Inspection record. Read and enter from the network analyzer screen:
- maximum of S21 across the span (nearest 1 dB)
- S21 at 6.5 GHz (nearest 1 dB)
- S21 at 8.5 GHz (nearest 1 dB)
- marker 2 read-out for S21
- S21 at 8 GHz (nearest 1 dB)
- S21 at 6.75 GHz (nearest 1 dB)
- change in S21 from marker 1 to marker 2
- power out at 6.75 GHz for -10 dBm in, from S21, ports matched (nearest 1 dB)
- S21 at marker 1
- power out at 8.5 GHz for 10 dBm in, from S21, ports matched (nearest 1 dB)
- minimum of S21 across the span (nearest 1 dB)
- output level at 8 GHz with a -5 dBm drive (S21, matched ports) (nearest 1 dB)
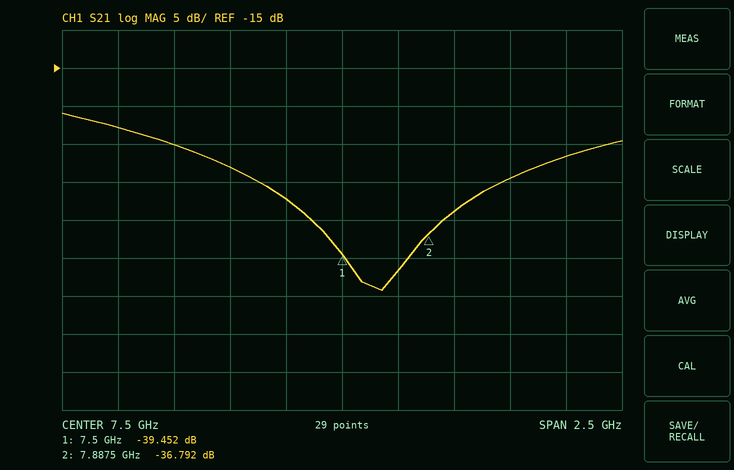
-21 dB
-23 dB
-27 dB
-36.792 dB
-34 dB
-25 dB
2.660 dB
-35 dBm
-39.452 dB
-17 dBm
-44 dB
-39 dBm
